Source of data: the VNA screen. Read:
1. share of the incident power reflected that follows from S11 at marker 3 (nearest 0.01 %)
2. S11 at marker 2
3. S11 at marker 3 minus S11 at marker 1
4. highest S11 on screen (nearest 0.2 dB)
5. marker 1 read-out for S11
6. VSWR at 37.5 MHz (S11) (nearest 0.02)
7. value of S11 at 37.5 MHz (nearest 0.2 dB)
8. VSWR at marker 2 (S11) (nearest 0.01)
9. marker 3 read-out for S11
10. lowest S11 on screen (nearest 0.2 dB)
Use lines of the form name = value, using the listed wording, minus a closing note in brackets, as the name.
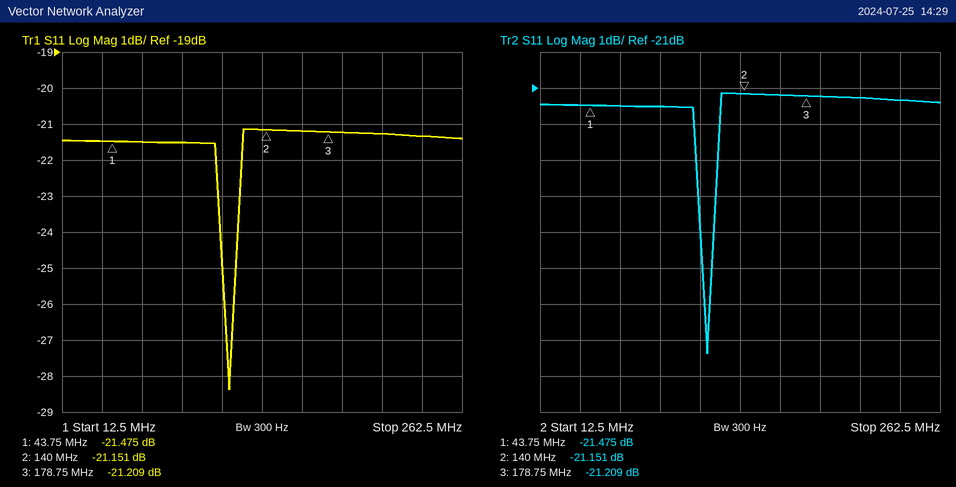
share of the incident power reflected that follows from S11 at marker 3 = 0.76 %
S11 at marker 2 = -21.151 dB
S11 at marker 3 minus S11 at marker 1 = 0.266 dB
highest S11 on screen = -21.2 dB
marker 1 read-out for S11 = -21.475 dB
VSWR at 37.5 MHz (S11) = 1.18
value of S11 at 37.5 MHz = -21.4 dB
VSWR at marker 2 (S11) = 1.19
marker 3 read-out for S11 = -21.209 dB
lowest S11 on screen = -28.4 dB
